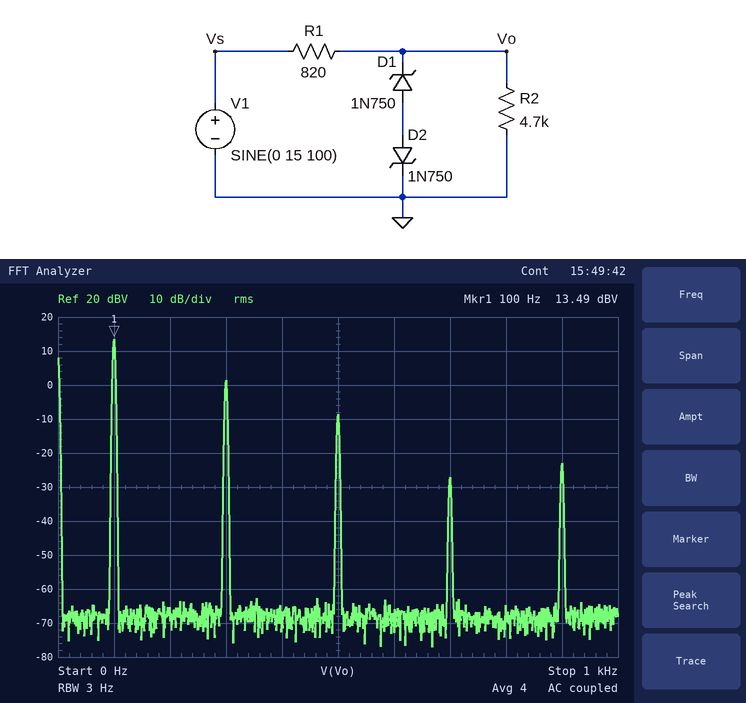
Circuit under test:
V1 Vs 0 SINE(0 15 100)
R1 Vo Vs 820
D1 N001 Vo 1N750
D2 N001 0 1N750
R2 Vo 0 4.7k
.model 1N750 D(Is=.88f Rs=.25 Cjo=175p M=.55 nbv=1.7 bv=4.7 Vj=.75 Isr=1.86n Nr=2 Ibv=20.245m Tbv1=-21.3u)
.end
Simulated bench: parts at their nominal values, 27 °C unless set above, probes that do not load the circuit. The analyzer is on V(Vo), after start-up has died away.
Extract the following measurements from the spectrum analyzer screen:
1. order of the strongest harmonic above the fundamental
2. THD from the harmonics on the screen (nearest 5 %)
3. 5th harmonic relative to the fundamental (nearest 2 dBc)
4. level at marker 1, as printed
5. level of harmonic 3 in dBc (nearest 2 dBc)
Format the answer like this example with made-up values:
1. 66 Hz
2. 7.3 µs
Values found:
1. 3
2. 25 %
3. -22 dBc
4. 13.49 dBV
5. -12 dBc
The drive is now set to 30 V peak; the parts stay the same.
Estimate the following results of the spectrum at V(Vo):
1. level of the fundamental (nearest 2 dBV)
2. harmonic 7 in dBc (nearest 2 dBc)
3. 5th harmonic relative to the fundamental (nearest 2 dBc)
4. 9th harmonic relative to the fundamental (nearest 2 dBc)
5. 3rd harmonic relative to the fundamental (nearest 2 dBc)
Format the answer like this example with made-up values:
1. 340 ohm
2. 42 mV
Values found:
1. 14 dBV
2. -20 dBc
3. -16 dBc
4. -26 dBc
5. -10 dBc
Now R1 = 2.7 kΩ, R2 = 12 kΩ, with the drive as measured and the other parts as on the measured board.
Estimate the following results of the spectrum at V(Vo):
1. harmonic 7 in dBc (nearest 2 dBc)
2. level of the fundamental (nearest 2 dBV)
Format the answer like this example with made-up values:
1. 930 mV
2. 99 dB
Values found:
1. -44 dBc
2. 14 dBV
